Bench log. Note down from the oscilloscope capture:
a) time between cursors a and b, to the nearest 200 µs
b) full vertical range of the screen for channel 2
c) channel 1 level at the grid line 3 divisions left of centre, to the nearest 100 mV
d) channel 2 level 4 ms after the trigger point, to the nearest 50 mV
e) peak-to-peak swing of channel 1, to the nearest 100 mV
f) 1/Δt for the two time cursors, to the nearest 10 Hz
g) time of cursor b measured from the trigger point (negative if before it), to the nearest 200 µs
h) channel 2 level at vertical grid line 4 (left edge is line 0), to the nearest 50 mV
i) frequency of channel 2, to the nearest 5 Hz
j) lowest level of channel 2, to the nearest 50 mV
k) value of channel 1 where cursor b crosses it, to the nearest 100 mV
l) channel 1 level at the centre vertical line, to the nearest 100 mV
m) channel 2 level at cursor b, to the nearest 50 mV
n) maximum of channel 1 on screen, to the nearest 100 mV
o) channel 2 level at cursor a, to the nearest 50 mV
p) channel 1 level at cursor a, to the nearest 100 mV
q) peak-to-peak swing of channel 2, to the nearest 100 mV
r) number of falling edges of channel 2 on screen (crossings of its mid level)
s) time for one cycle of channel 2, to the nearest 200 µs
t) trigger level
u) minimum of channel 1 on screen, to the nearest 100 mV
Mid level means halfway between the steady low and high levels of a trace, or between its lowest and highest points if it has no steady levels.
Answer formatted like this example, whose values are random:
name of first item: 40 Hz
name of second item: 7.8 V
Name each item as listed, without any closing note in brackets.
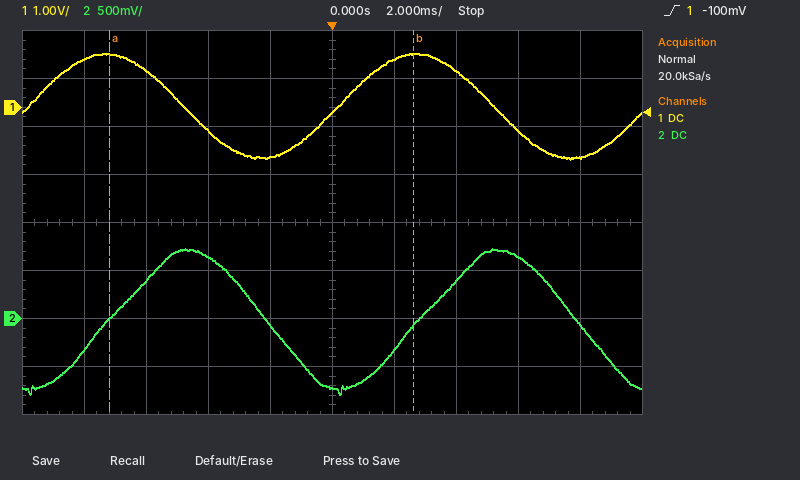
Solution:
time between cursors a and b, to the nearest 200 µs: 9.8 ms
full vertical range of the screen for channel 2: 4 V
channel 1 level at the grid line 3 divisions left of centre, to the nearest 100 mV: 800 mV
channel 2 level 4 ms after the trigger point, to the nearest 50 mV: 400 mV
peak-to-peak swing of channel 1, to the nearest 100 mV: 2.2 V
1/Δt for the two time cursors, to the nearest 10 Hz: 100 Hz
time of cursor b measured from the trigger point (negative if before it), to the nearest 200 µs: +2.6 ms
channel 2 level at vertical grid line 4 (left edge is line 0), to the nearest 50 mV: -50 mV
frequency of channel 2, to the nearest 5 Hz: 100 Hz
lowest level of channel 2, to the nearest 50 mV: -800 mV
value of channel 1 where cursor b crosses it, to the nearest 100 mV: 1.1 V
channel 1 level at the centre vertical line, to the nearest 100 mV: -100 mV
channel 2 level at cursor b, to the nearest 50 mV: -50 mV
maximum of channel 1 on screen, to the nearest 100 mV: 1.1 V
channel 2 level at cursor a, to the nearest 50 mV: 0 mV
channel 1 level at cursor a, to the nearest 100 mV: 1.1 V
peak-to-peak swing of channel 2, to the nearest 100 mV: 1.50 V
number of falling edges of channel 2 on screen: 2
time for one cycle of channel 2, to the nearest 200 µs: 10.0 ms
trigger level: -100 mV
minimum of channel 1 on screen, to the nearest 100 mV: -1.1 V
